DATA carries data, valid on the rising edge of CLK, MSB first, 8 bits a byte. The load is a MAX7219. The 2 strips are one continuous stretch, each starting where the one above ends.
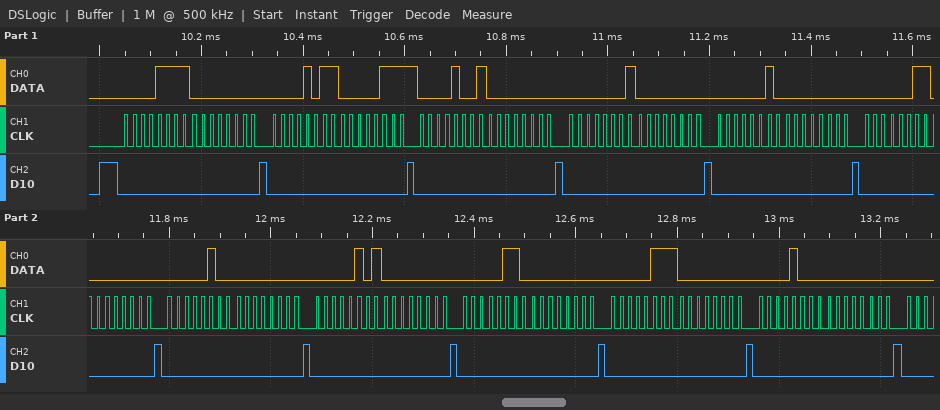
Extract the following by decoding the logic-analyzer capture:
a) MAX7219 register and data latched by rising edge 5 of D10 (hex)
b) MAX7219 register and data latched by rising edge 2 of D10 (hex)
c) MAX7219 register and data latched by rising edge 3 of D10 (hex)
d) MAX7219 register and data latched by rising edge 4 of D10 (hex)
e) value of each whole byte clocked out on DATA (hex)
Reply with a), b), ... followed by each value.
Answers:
a) register 0x1, data 0x00
b) register 0xF, data 0x00
c) register 0xB, data 0x07
d) register 0x9, data 0x00
e) 0x0F 0x00 0x0B 0x07 0x09 0x00 0x01 0x00 0x02 0x00 0x03 0x00 0x04 0x00 0x05 0x00 0x06 0x00 0x07 0x00 0x08 0x00
